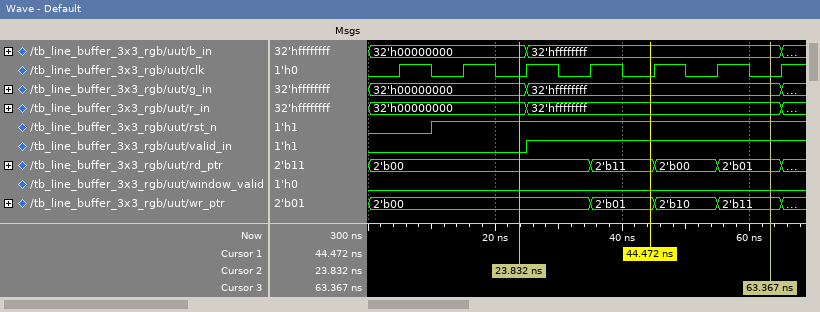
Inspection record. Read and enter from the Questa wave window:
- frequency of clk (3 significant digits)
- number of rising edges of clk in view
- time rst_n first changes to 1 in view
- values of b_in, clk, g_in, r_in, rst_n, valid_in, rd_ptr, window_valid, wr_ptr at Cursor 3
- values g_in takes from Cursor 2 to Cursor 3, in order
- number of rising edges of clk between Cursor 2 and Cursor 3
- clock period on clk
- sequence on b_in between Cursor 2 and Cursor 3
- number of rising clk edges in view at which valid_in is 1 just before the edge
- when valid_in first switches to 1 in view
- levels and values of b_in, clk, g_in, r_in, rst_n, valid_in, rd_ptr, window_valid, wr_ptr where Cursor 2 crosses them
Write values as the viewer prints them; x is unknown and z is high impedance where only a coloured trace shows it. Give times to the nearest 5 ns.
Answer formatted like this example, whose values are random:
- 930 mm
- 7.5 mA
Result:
- 100 MHz
- 7
- 10 ns
- b_in=32'hffffffff, clk=0, g_in=32'hffffffff, r_in=32'hffffffff, rst_n=1, valid_in=1, rd_ptr=2'b01, window_valid=0, wr_ptr=2'b11
- 32'h00000000, 32'hffffffff
- 4
- 10 ns
- 32'h00000000, 32'hffffffff
- 4
- 25 ns
- b_in=32'h00000000, clk=0, g_in=32'h00000000, r_in=32'h00000000, rst_n=1, valid_in=0, rd_ptr=2'b00, window_valid=0, wr_ptr=2'b00
